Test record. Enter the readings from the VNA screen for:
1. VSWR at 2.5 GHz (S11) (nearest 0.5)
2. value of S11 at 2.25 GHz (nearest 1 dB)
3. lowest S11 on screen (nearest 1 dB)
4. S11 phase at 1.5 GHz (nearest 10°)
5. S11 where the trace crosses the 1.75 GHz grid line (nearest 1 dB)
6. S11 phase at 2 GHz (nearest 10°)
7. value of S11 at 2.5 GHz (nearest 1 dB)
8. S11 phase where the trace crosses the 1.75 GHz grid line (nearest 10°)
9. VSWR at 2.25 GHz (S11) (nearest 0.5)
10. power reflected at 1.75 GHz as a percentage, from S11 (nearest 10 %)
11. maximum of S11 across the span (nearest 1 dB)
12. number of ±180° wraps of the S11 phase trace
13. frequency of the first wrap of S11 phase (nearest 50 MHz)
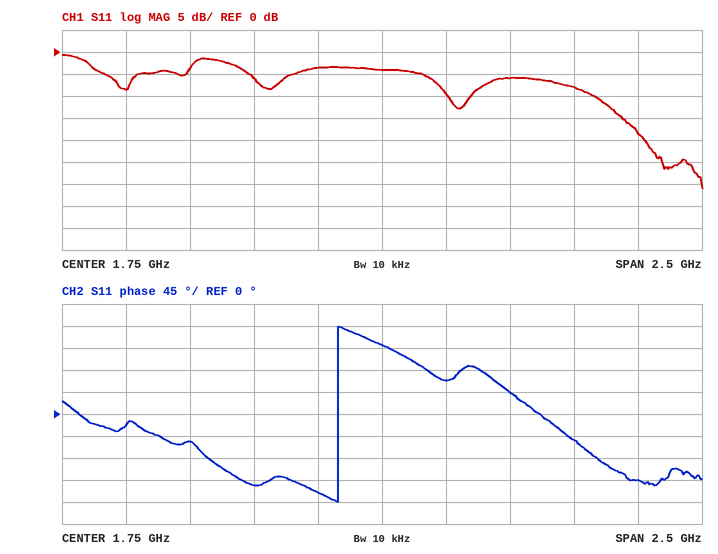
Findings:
2.5
-6 dB
-31 dB
-160°
-4 dB
70°
-8 dB
140°
3.0
40 %
-1 dB
1
1.60 GHz
